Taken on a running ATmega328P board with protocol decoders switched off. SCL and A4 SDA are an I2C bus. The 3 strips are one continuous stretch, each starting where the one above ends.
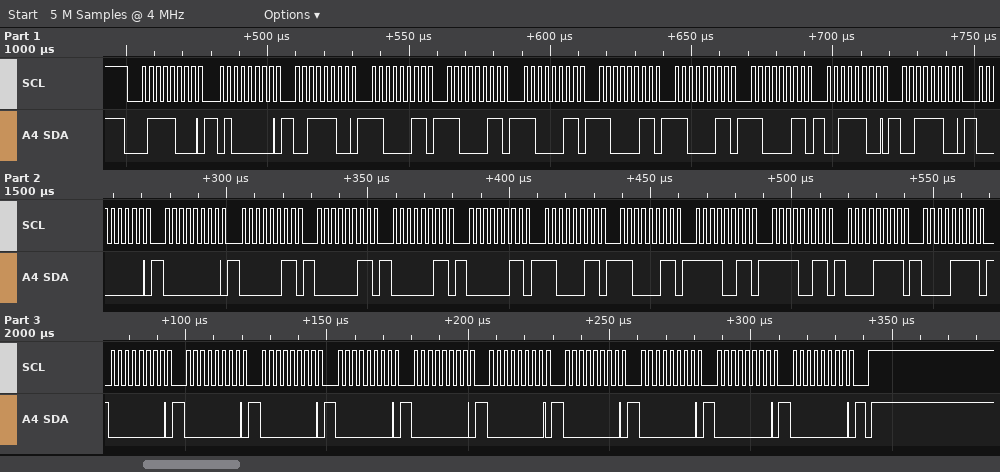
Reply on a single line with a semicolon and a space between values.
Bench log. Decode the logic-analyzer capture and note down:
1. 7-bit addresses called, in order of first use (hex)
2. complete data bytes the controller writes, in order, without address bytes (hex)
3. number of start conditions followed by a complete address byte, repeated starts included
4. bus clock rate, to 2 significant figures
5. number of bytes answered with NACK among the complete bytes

0x3C; 40 3C C3 C3 C3 C3 C3 C3 3C 3C 00 00 03 03 03 03 C3 C3 F3 F3 0F 0F 00 00 00 00 00 00 00 00 00 00; 1; 400 kHz; 0
